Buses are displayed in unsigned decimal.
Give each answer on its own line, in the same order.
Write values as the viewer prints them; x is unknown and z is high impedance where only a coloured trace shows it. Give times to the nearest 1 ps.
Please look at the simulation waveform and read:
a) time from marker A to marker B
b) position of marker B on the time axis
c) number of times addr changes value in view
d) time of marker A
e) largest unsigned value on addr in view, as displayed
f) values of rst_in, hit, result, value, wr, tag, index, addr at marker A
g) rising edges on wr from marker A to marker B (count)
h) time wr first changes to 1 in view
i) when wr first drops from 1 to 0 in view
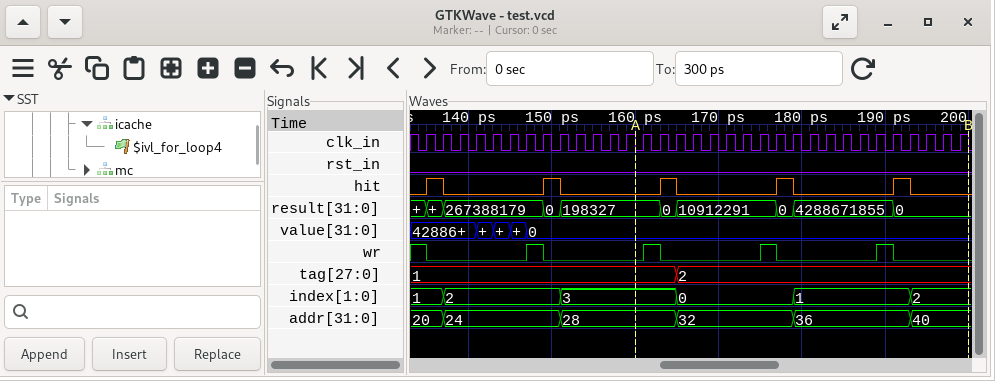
40 ps
200 ps
5
160 ps
40
rst_in=0, hit=0, result=198327, value=0, wr=0, tag=1, index=3, addr=28
3
147 ps
135 ps
